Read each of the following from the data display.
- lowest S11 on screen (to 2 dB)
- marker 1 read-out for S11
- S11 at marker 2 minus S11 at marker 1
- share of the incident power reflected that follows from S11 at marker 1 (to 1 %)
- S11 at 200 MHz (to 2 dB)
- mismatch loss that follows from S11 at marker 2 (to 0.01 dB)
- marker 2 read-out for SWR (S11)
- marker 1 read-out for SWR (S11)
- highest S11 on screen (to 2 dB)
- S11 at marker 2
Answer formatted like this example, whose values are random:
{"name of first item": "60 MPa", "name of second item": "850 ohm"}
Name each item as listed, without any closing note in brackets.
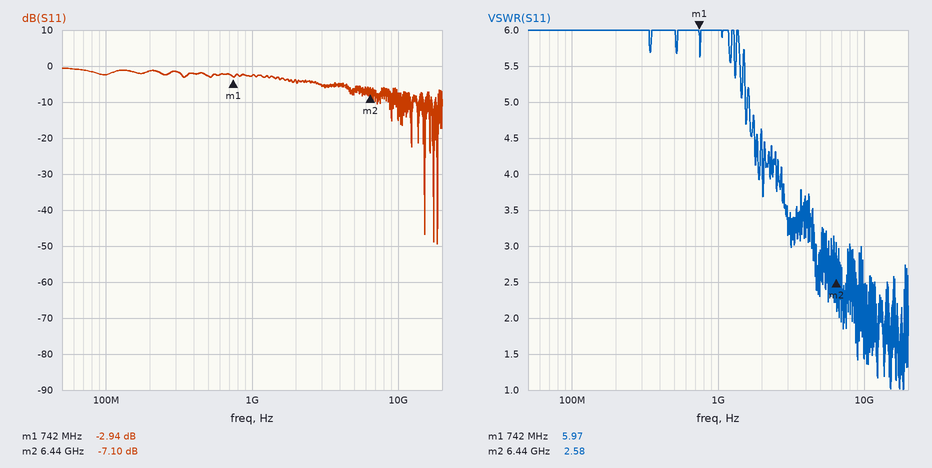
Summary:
{"lowest S11 on screen": "-50 dB", "marker 1 read-out for S11": "-2.94 dB", "S11 at marker 2 minus S11 at marker 1": "-4.16 dB", "share of the incident power reflected that follows from S11 at marker 1": "51 %", "S11 at 200 MHz": "-2 dB", "mismatch loss that follows from S11 at marker 2": "0.94 dB", "marker 2 read-out for SWR": "2.58", "marker 1 read-out for SWR": "5.97", "highest S11 on screen": "0 dB", "S11 at marker 2": "-7.10 dB"}
